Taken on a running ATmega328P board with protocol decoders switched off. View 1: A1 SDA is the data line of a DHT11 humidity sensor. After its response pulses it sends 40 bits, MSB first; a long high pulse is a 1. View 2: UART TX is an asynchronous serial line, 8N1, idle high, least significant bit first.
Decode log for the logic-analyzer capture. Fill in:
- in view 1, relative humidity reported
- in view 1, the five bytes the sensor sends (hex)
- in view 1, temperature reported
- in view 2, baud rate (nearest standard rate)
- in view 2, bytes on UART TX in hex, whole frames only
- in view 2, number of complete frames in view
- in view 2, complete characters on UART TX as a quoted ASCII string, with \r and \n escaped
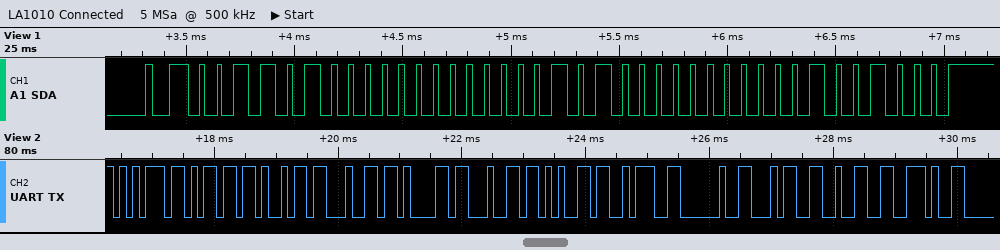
52 %
34 00 14 00 48
20.0 °C
9600 baud
75 6D 69 64 61 64 65 3A 20 34 32 2E
12
"umidade: 42."
